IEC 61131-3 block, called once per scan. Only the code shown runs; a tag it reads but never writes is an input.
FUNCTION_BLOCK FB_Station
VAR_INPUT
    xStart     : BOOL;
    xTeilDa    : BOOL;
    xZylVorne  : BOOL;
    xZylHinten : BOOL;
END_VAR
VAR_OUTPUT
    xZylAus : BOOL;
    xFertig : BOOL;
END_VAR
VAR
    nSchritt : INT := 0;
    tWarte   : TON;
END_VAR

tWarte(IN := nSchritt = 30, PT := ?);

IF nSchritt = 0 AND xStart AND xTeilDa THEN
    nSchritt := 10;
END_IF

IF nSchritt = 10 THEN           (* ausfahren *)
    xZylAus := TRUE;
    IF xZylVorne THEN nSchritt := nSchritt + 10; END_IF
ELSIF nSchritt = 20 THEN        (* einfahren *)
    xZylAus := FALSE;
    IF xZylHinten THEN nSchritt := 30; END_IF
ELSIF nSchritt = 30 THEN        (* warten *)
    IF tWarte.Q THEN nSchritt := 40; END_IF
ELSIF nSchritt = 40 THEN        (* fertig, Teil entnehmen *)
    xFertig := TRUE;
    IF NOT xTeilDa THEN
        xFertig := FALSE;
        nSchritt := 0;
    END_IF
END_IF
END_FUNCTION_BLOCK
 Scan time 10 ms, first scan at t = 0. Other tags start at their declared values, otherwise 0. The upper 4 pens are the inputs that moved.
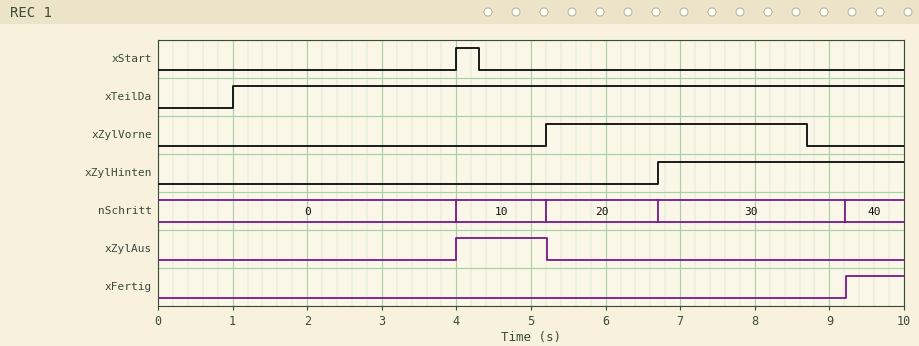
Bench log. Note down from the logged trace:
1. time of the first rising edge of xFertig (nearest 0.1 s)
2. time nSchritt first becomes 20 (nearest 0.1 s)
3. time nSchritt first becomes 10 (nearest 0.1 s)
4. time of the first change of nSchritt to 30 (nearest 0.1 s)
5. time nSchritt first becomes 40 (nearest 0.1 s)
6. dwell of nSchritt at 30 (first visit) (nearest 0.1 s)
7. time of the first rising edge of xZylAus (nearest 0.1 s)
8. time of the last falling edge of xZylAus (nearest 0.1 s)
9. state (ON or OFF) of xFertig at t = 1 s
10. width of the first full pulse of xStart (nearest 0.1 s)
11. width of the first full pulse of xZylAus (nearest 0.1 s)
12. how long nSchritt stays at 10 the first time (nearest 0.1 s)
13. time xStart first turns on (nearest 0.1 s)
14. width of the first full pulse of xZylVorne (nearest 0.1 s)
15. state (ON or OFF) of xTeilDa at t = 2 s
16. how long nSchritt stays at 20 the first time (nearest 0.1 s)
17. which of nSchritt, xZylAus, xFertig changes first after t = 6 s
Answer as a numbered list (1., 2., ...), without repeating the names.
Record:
1. 9.2 s
2. 5.2 s
3. 4.0 s
4. 6.7 s
5. 9.2 s
6. 2.5 s
7. 4.0 s
8. 5.2 s
9. OFF
10. 0.3 s
11. 1.2 s
12. 1.2 s
13. 4.0 s
14. 3.5 s
15. ON
16. 1.5 s
17. nSchritt
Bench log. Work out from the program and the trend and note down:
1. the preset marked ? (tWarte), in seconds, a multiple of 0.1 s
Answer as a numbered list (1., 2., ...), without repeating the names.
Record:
1. 2.5 s
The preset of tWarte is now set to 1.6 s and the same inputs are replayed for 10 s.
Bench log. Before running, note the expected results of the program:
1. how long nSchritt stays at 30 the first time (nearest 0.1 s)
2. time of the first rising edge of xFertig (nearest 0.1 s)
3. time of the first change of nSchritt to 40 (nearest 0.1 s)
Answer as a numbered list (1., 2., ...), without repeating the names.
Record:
1. 1.6 s
2. 8.3 s
3. 8.3 s
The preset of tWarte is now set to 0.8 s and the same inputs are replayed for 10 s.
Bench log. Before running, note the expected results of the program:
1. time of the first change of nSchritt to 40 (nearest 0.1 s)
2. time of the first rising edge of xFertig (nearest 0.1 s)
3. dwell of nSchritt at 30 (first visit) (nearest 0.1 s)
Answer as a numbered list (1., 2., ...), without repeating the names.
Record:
1. 7.5 s
2. 7.5 s
3. 0.8 s
